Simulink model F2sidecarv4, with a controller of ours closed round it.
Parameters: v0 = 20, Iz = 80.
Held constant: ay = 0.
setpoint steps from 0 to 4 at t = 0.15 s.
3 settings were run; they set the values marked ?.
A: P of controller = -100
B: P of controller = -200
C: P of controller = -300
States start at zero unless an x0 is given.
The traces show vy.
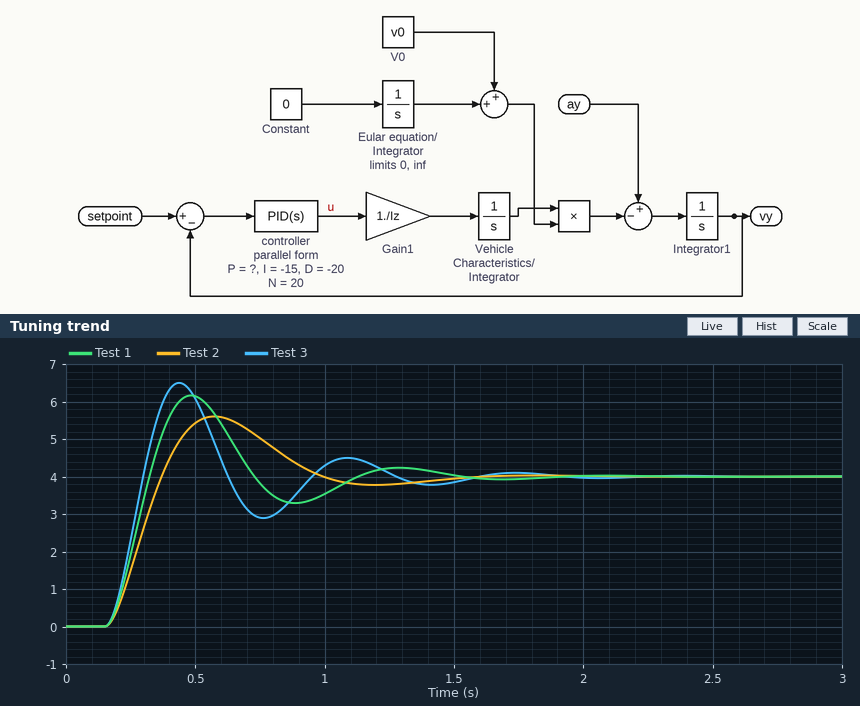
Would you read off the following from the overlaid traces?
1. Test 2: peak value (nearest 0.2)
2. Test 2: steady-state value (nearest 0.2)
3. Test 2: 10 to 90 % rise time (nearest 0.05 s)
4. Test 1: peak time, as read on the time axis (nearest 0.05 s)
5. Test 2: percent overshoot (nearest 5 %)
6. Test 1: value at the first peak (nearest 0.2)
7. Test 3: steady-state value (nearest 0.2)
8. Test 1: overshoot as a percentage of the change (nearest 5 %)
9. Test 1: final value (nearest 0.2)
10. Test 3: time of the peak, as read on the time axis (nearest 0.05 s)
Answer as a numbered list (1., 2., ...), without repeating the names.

1. 5.6
2. 4.0
3. 0.15 s
4. 0.50 s
5. 40 %
6. 6.2
7. 4.0
8. 55 %
9. 4.0
10. 0.45 s
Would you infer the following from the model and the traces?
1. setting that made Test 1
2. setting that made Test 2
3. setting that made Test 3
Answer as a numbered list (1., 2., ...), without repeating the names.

1. B
2. A
3. C
